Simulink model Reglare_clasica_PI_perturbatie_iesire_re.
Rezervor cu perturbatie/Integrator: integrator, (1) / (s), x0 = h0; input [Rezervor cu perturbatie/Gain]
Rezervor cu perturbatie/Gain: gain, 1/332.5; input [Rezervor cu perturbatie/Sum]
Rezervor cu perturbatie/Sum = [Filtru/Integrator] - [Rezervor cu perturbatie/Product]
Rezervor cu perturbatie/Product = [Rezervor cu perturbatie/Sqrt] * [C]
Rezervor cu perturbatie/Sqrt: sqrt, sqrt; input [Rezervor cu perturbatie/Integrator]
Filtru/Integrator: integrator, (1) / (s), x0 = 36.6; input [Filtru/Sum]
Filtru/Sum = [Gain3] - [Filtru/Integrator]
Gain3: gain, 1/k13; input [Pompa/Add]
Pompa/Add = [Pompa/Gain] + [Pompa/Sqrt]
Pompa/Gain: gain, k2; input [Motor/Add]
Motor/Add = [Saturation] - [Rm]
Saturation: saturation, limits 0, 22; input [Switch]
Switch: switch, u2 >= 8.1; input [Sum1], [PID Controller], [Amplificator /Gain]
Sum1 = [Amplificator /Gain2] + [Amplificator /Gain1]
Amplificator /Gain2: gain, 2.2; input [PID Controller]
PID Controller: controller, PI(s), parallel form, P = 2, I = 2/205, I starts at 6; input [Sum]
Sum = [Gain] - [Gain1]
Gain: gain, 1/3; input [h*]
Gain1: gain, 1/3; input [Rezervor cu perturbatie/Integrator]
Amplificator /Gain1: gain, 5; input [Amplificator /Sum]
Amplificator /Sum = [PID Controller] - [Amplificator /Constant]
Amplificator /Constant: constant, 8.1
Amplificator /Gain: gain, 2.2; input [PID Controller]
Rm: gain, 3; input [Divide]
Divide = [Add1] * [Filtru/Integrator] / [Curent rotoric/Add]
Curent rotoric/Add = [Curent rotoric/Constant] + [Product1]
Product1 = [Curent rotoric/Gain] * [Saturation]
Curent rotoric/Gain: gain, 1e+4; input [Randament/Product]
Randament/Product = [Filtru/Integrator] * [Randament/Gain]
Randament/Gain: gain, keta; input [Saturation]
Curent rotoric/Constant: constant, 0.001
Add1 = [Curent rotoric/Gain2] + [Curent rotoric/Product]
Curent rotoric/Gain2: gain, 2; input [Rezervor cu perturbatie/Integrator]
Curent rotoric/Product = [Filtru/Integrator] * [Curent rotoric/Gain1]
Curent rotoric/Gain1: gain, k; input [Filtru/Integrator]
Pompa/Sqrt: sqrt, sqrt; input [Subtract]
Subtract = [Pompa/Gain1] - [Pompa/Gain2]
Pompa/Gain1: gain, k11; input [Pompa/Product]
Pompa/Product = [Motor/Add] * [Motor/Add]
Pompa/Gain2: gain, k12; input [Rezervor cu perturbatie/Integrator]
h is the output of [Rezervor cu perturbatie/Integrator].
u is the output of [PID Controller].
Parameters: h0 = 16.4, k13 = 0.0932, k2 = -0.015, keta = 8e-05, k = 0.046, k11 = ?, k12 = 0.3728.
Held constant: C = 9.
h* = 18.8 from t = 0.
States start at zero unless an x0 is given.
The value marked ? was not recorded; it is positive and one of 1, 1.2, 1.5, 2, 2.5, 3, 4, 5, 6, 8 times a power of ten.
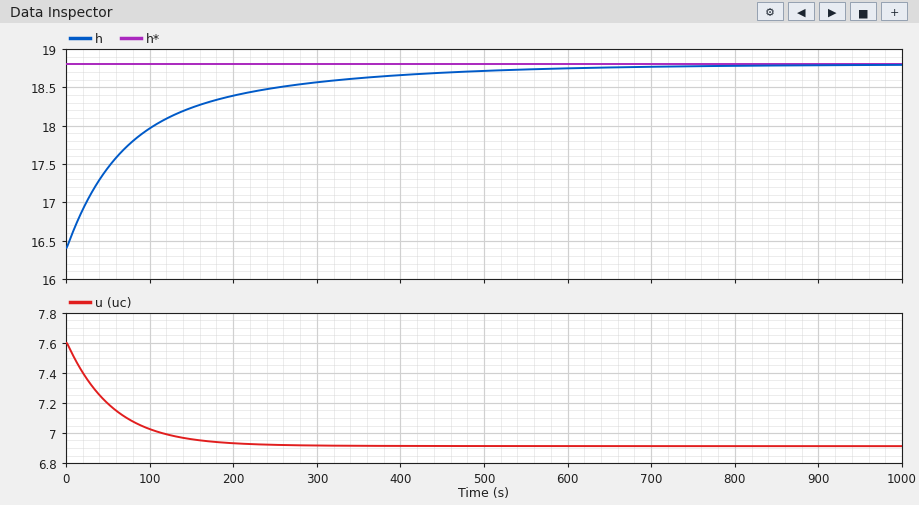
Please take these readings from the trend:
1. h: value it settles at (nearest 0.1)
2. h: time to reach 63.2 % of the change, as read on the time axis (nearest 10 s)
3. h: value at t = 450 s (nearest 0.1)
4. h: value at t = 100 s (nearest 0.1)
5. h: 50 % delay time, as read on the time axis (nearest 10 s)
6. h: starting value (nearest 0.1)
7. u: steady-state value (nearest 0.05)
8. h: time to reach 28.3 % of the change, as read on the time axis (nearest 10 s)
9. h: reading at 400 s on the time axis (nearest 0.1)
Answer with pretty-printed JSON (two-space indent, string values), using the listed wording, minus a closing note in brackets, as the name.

{
  "h: value it settles at": "18.8",
  "h: time to reach 63.2 % of the change, as read on the time axis": "90 s",
  "h: value at t = 450 s": "18.7",
  "h: value at t = 100 s": "18.0",
  "h: 50 % delay time, as read on the time axis": "60 s",
  "h: starting value": "16.4",
  "u: steady-state value": "6.90",
  "h: time to reach 28.3 % of the change, as read on the time axis": "30 s",
  "h: reading at 400 s on the time axis": "18.7"
}
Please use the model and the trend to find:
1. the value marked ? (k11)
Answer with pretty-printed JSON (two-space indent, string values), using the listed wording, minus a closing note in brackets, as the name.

{
  "the value marked ?": "0.12"
}
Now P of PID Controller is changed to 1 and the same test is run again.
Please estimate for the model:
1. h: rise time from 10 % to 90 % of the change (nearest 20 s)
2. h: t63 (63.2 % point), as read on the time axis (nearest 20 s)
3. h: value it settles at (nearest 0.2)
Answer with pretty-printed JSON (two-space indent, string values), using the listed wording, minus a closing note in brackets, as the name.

{
  "h: rise time from 10 % to 90 % of the change": "220 s",
  "h: t63 (63.2 % point), as read on the time axis": "140 s",
  "h: value it settles at": "18.8"
}
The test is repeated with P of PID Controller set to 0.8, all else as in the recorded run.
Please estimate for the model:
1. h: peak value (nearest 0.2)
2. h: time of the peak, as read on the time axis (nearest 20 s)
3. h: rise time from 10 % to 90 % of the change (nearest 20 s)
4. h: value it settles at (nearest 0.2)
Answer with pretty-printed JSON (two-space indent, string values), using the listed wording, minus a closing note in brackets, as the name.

{
  "h: peak value": "19.0",
  "h: time of the peak, as read on the time axis": "400 s",
  "h: rise time from 10 % to 90 % of the change": "200 s",
  "h: value it settles at": "18.8"
}
